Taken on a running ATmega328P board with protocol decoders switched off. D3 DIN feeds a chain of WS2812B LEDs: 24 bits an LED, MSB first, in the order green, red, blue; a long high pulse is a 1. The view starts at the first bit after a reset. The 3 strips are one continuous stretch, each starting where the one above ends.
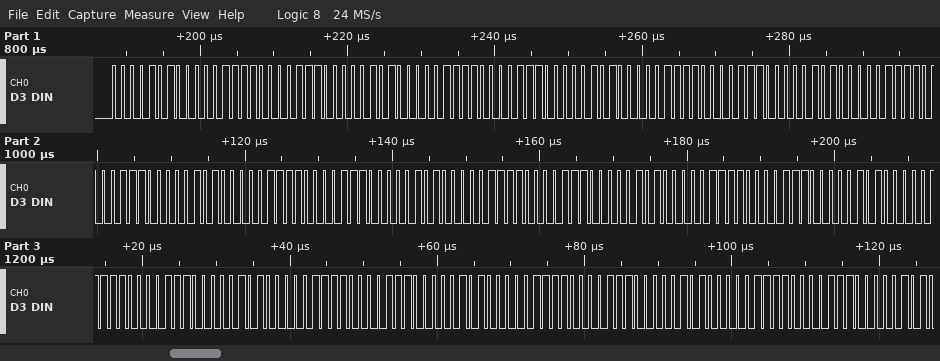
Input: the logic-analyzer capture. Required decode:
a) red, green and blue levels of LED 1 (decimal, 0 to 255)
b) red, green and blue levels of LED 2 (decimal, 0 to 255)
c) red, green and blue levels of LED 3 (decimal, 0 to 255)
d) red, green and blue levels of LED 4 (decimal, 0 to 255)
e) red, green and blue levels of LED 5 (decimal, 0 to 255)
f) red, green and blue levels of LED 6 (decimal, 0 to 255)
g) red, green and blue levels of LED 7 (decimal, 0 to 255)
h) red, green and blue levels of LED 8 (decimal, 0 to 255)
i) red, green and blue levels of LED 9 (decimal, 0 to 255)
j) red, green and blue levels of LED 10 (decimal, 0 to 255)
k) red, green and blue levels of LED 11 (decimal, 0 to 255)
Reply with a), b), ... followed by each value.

a) 15, 10, 14
b) 15, 10, 14
c) 15, 10, 14
d) 15, 10, 14
e) 15, 10, 14
f) 15, 10, 14
g) 15, 10, 14
h) 15, 10, 14
i) 15, 10, 14
j) 15, 10, 14
k) 15, 10, 14
